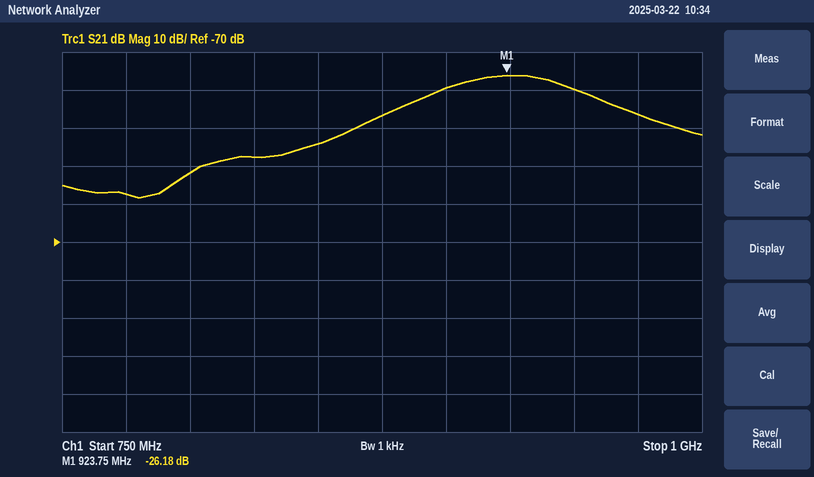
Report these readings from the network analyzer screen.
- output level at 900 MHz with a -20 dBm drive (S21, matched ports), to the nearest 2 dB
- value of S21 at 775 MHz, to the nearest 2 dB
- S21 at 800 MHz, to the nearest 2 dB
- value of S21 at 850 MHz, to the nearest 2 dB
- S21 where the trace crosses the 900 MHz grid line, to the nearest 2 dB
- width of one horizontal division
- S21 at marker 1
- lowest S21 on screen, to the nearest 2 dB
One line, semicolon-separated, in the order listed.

-50 dBm; -58 dB; -52 dB; -44 dB; -30 dB; 25 MHz; -26.18 dB; -58 dB
